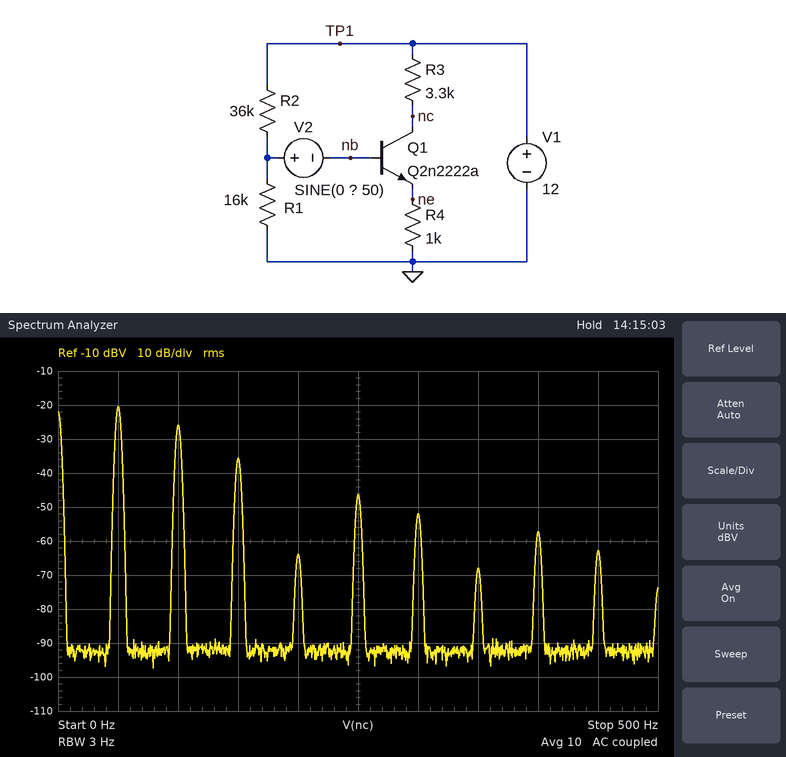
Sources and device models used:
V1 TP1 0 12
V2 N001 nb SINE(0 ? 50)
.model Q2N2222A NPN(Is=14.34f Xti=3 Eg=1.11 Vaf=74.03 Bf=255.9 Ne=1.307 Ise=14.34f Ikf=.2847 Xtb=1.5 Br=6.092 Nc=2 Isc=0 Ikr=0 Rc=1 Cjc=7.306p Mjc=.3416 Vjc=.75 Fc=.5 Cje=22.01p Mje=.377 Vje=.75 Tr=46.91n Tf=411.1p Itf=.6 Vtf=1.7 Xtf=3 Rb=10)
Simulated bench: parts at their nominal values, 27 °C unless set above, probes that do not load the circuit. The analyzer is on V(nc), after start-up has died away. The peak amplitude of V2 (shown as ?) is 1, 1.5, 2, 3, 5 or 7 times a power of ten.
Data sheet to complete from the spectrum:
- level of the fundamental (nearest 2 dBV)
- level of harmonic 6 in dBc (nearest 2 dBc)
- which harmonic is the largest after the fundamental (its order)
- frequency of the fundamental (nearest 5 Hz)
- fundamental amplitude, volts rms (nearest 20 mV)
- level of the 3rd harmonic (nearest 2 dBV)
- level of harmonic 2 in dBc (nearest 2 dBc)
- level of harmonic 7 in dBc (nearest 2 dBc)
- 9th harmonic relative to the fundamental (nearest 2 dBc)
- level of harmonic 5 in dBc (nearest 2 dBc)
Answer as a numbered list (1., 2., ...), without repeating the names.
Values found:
1. -20 dBV
2. -32 dBc
3. 2
4. 50 Hz
5. 100 mV
6. -36 dBV
7. -6 dBc
8. -48 dBc
9. -42 dBc
10. -26 dBc
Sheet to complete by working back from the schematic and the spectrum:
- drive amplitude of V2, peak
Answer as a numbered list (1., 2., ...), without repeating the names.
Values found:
1. 150 mV
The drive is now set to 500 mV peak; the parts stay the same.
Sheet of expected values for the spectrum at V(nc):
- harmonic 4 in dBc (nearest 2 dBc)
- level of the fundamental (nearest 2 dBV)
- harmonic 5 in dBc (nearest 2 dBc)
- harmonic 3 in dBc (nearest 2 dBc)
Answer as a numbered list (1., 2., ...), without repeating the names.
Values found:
1. -22 dBc
2. -6 dBV
3. -32 dBc
4. -26 dBc
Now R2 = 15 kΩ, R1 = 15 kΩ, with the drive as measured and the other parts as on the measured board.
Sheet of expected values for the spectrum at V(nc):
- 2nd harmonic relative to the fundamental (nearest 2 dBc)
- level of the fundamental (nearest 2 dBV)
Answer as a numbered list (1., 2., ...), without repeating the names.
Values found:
1. -58 dBc
2. -40 dBV
